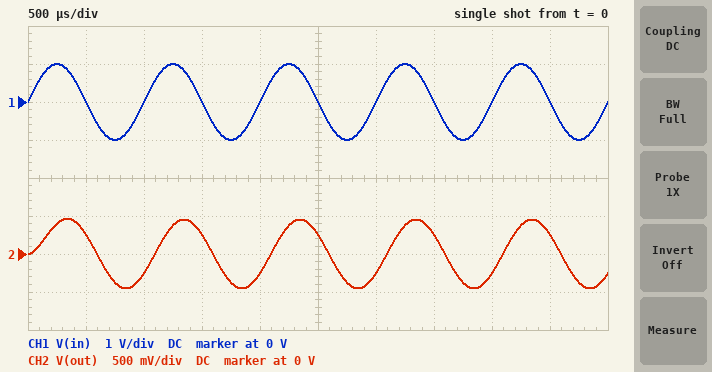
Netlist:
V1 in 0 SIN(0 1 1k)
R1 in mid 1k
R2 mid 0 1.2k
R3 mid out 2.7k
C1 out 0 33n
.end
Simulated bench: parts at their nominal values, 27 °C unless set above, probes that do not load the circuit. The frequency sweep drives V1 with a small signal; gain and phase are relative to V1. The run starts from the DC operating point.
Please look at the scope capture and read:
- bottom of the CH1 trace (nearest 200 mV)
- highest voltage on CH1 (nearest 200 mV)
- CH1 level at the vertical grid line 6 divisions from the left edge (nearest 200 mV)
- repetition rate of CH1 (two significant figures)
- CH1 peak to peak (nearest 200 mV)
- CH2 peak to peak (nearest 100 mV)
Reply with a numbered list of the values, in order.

1. -1.0 V
2. 1.0 V
3. 0 V
4. 1.0 kHz
5. 2.0 V
6. 900 mV
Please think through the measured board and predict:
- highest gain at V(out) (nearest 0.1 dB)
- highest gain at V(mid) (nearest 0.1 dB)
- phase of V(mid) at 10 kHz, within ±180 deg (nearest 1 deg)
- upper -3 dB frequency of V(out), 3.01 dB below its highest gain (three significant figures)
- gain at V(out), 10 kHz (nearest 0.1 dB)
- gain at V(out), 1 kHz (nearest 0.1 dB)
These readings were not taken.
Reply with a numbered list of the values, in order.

1. -5.3 dB
2. -5.3 dB
3. -2 deg
4. 1.49 kHz
5. -21.9 dB
6. -6.9 dB
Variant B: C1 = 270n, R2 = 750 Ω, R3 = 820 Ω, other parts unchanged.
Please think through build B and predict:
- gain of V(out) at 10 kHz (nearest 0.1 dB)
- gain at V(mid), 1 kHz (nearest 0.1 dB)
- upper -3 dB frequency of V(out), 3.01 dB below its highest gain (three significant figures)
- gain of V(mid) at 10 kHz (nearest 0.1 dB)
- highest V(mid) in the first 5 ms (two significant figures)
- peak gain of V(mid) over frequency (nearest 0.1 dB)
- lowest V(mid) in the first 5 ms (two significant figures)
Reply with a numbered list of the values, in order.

1. -33.9 dB
2. -10.1 dB
3. 472 Hz
4. -11.0 dB
5. 340 mV
6. -7.4 dB
7. -310 mV
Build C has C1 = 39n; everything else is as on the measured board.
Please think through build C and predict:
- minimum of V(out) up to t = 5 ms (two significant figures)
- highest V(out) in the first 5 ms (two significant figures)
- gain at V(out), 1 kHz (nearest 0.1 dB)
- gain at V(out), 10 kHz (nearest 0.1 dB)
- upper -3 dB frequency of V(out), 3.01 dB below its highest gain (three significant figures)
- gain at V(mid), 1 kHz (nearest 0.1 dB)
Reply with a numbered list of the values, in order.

1. -430 mV
2. 440 mV
3. -7.4 dB
4. -23.3 dB
5. 1.26 kHz
6. -5.8 dB
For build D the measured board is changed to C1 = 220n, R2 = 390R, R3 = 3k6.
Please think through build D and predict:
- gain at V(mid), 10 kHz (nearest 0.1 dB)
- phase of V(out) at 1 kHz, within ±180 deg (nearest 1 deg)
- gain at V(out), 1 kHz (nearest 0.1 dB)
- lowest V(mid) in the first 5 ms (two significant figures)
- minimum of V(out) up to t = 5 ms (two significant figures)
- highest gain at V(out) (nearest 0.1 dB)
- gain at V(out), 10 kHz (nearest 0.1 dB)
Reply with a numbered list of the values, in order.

1. -11.7 dB
2. -79 deg
3. -25.8 dB
4. -260 mV
5. -51 mV
6. -11.0 dB
7. -45.6 dB
